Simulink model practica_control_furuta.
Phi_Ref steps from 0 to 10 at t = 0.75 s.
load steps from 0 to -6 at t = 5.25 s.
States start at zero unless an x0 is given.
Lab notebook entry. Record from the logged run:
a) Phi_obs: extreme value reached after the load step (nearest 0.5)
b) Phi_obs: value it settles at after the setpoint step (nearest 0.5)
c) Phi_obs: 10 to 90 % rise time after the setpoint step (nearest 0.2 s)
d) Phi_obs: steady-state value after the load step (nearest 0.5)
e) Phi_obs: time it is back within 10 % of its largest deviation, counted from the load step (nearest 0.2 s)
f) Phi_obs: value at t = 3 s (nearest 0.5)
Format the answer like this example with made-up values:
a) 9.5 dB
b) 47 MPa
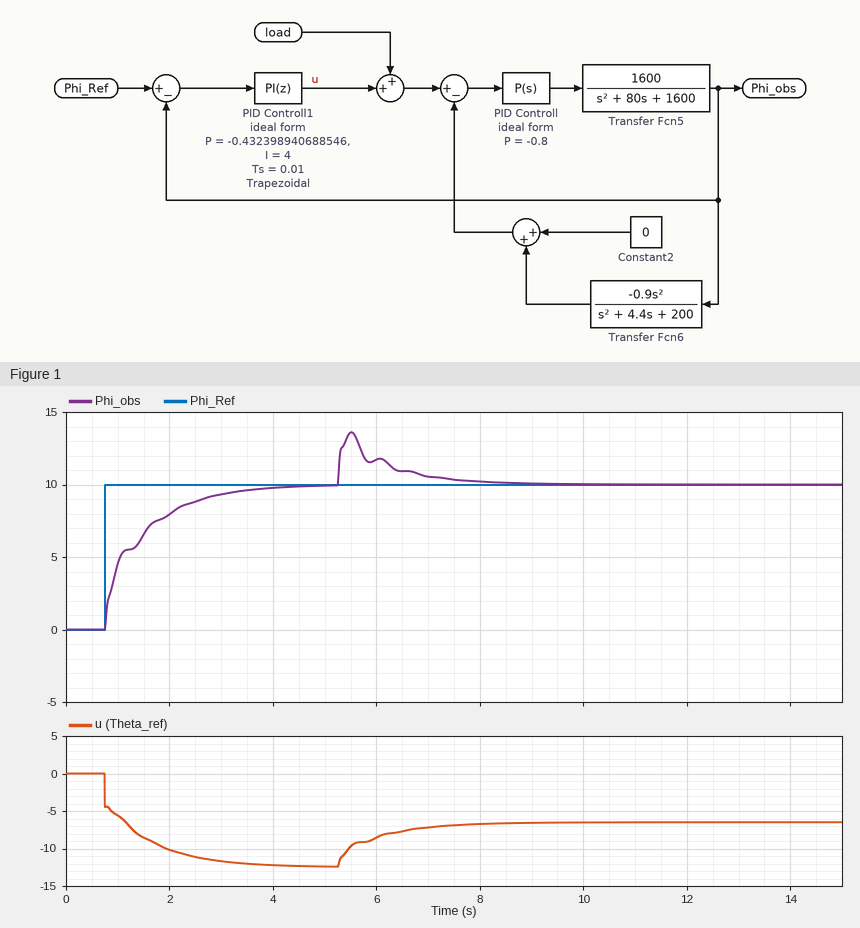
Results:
a) 13.5
b) 10.0
c) 1.8 s
d) 10.0
e) 2.2 s
f) 9.5
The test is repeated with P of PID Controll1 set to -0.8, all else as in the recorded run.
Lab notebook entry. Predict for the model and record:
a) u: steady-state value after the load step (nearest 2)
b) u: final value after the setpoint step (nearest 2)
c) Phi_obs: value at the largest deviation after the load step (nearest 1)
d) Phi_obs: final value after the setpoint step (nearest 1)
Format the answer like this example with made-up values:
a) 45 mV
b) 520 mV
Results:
a) -6
b) -12
c) 13
d) 10
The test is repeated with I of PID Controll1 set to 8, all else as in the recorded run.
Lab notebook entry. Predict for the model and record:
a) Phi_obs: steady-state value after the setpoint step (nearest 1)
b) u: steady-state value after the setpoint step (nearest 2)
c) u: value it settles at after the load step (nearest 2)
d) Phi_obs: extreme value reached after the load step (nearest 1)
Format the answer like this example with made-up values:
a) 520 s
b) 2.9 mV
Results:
a) 10
b) -12
c) -6
d) 13
